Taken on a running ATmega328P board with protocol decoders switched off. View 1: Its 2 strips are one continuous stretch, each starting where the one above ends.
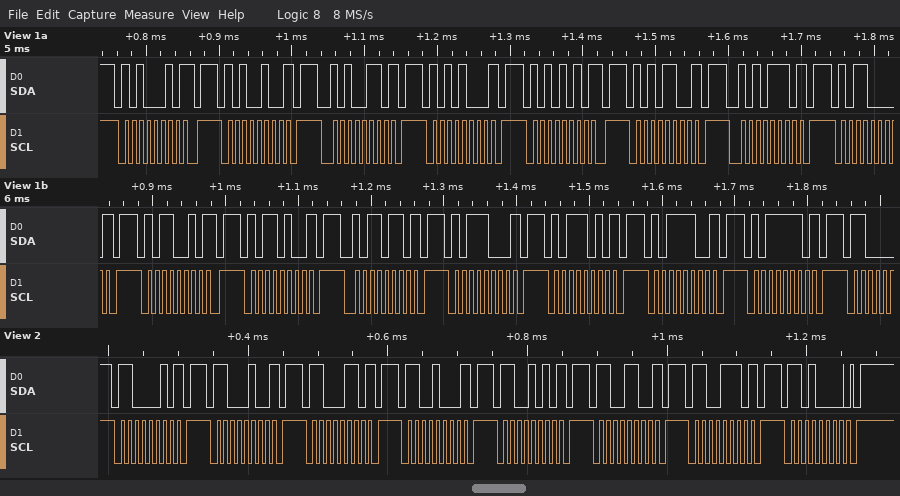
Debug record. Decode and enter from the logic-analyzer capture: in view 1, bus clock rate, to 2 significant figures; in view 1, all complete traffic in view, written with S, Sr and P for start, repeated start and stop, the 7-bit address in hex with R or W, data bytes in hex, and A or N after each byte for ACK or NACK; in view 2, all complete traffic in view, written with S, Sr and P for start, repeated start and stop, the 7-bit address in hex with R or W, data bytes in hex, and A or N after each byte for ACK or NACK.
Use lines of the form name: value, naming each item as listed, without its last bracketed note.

in view 1, bus clock rate, to 2 significant figures: 100 kHz
in view 1, all complete traffic in view, written with S, Sr and P for start, repeated start and stop, the 7-bit address in hex with R or W, data bytes in hex, and A or N after each byte for ACK or NACK: S 51W N P S 52W N P S 53W N P S 54W N P S 55W N P S 56W N P S 57W N P S 58W N P S 59W N P S 5AW N P S 5BW N P S 5CW N P S 5DW N P S 5EW N P S 5FW N P
in view 2, all complete traffic in view, written with S, Sr and P for start, repeated start and stop, the 7-bit address in hex with R or W, data bytes in hex, and A or N after each byte for ACK or NACK: S 61W N P S 62W N P S 63W N P S 64W N P S 65W N P S 66W N P S 67W N P S 68W A P
